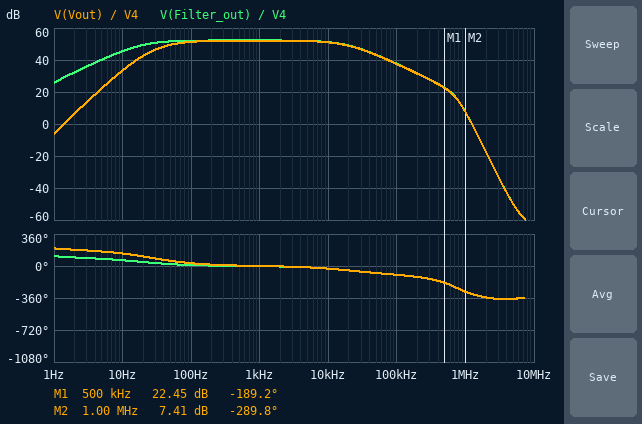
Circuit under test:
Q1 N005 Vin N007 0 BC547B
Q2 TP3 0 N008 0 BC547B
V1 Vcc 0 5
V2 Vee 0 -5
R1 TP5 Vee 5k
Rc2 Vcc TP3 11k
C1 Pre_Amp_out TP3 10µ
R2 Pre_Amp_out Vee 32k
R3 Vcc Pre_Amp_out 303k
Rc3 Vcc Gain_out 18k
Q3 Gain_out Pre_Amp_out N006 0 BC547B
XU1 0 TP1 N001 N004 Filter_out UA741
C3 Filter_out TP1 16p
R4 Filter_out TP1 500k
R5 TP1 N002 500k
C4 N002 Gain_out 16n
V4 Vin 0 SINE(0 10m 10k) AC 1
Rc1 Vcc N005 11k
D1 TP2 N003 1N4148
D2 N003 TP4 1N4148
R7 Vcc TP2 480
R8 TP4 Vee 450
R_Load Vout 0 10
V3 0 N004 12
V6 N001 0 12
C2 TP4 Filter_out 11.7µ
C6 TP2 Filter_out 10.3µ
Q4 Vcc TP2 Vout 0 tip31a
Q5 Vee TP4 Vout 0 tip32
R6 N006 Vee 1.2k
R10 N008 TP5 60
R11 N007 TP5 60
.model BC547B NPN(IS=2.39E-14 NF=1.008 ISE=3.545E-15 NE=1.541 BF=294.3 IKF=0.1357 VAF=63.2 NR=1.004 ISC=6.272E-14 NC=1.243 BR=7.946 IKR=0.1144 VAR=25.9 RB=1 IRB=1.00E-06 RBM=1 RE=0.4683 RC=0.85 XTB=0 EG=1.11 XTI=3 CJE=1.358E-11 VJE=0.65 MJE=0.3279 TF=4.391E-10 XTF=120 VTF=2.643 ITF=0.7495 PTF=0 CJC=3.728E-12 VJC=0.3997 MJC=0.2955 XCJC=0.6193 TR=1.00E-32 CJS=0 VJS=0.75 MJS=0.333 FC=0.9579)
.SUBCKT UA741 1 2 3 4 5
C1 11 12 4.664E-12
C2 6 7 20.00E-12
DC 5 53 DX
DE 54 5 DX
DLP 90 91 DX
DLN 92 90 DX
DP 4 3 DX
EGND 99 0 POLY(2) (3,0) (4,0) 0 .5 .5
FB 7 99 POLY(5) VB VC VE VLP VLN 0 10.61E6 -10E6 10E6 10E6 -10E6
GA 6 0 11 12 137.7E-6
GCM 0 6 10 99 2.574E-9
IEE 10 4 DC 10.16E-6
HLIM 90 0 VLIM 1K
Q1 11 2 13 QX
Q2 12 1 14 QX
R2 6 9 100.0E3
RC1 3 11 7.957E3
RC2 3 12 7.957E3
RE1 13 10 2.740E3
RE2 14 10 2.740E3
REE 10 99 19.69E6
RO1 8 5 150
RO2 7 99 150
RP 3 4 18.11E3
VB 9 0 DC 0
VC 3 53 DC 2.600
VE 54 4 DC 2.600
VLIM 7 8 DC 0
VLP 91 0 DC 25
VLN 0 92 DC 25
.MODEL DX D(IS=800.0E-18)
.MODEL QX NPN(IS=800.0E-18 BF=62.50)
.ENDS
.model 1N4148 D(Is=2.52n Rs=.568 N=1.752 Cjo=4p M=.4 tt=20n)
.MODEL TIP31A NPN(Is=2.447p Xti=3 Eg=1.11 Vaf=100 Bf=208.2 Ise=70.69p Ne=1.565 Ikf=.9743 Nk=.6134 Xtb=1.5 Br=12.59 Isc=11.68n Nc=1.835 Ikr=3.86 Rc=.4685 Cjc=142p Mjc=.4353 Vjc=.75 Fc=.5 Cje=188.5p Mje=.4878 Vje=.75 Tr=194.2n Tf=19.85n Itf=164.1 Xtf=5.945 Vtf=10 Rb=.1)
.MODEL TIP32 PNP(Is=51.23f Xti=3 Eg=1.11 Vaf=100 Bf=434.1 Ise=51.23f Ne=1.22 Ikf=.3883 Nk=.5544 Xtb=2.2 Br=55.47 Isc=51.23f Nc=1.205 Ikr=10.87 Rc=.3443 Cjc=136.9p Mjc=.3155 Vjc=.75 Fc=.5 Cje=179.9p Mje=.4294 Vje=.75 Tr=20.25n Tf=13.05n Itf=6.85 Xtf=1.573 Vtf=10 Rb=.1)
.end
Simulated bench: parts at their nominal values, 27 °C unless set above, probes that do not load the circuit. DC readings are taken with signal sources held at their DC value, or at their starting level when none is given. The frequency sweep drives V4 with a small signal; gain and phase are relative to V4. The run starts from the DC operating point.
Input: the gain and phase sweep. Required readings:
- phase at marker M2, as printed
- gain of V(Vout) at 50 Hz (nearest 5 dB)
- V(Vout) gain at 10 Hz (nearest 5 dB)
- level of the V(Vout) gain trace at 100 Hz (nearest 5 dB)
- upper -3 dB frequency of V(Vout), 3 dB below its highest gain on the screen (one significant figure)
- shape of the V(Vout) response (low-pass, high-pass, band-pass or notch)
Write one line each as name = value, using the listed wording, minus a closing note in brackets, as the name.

phase at marker M2, as printed = -289.8 deg
gain of V(Vout) at 50 Hz = 50 dB
V(Vout) gain at 10 Hz = 35 dB
level of the V(Vout) gain trace at 100 Hz = 50 dB
upper -3 dB frequency of V(Vout), 3 dB below its highest gain on the screen = 20 kHz
shape of the V(Vout) response = band-pass
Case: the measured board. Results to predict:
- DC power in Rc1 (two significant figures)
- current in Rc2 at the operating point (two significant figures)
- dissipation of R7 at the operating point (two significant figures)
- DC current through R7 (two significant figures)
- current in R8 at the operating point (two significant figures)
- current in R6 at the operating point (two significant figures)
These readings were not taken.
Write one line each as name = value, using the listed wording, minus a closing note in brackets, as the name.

DC power in Rc1 = 2.1 mW
current in Rc2 at the operating point = 430 µA
dissipation of R7 at the operating point = 41 mW
DC current through R7 = 9.2 mA
current in R8 at the operating point = 9.3 mA
current in R6 at the operating point = 270 µA
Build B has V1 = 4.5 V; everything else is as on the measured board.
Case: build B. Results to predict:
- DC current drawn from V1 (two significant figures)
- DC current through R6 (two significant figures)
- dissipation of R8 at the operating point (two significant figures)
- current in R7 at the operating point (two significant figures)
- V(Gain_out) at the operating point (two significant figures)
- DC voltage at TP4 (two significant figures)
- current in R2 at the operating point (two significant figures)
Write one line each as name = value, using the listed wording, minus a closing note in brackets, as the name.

DC current drawn from V1 = 85 mA
DC current through R6 = 240 µA
dissipation of R8 at the operating point = 36 mW
current in R7 at the operating point = 8.6 mA
V(Gain_out) at the operating point = 230 mV
DC voltage at TP4 = -1.0 V
current in R2 at the operating point = 28 µA
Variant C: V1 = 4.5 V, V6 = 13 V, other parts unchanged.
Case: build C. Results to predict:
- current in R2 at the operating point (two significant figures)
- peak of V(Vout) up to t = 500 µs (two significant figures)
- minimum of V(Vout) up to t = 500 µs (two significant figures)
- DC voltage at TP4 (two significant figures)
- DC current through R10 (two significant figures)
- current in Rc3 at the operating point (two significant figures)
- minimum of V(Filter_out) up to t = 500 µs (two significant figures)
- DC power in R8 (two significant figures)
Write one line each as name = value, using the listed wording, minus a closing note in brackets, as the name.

current in R2 at the operating point = 28 µA
peak of V(Vout) up to t = 500 µs = 2.6 V
minimum of V(Vout) up to t = 500 µs = -3.1 V
DC voltage at TP4 = -1.0 V
DC current through R10 = 440 µA
current in Rc3 at the operating point = 240 µA
minimum of V(Filter_out) up to t = 500 µs = -2.8 V
DC power in R8 = 36 mW
